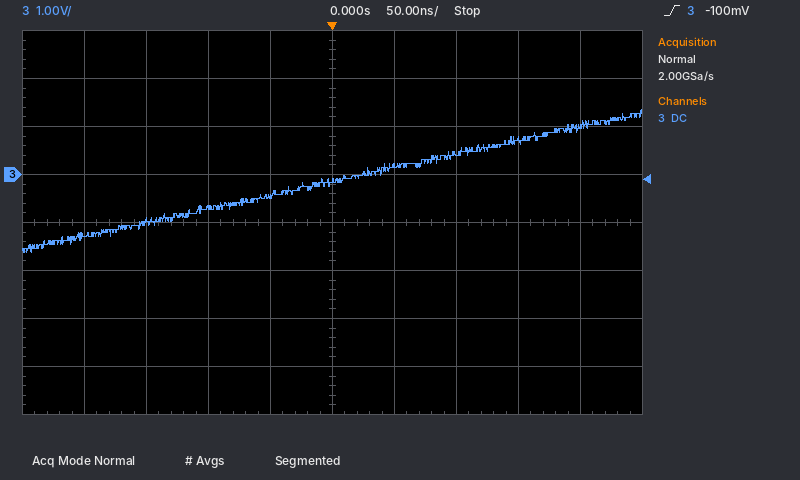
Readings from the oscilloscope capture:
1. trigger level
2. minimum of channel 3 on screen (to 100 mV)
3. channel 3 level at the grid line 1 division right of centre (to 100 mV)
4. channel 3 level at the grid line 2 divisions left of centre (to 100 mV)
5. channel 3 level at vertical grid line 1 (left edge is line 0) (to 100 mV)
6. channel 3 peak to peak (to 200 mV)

-100 mV
-1.6 V
200 mV
-700 mV
-1.3 V
3.0 V
